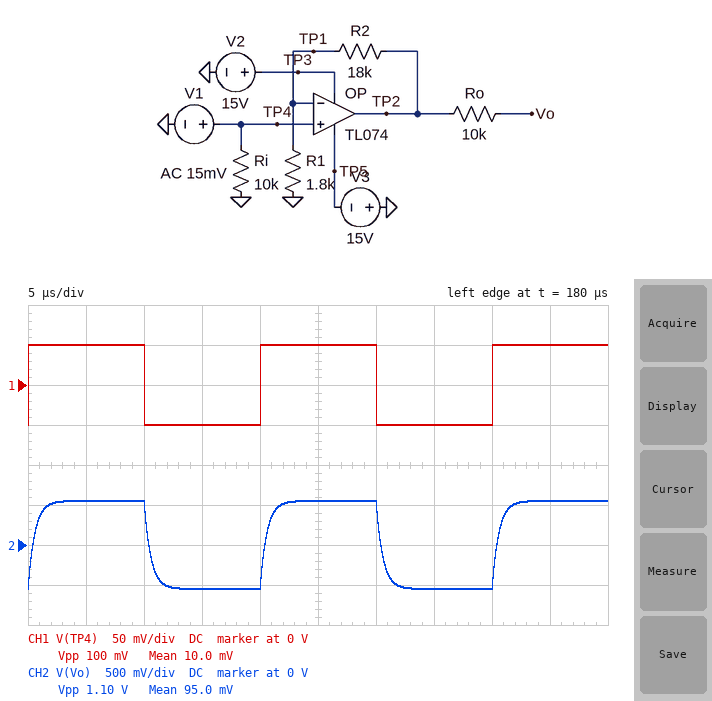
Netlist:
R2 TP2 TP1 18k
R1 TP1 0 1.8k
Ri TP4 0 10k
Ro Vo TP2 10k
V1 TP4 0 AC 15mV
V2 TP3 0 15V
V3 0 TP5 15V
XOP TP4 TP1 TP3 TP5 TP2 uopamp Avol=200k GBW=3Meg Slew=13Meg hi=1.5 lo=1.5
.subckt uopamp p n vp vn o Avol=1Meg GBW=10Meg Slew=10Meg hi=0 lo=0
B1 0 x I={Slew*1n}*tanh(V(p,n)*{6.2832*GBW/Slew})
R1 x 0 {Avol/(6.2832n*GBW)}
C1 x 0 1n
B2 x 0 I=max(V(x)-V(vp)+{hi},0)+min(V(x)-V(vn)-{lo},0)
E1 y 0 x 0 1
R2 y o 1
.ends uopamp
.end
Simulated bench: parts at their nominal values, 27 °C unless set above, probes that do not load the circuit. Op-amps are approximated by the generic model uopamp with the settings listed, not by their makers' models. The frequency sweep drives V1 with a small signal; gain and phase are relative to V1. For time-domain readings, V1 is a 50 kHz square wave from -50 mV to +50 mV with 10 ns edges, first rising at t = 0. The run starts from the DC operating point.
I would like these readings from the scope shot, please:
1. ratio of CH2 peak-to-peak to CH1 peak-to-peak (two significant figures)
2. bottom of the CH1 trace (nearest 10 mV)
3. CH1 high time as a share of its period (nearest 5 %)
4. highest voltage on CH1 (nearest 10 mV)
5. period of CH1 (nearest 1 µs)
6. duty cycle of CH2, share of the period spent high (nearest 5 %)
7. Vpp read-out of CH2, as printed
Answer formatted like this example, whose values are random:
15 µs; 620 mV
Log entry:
11; -50 mV; 50 %; 50 mV; 20 µs; 50 %; 1.10 V
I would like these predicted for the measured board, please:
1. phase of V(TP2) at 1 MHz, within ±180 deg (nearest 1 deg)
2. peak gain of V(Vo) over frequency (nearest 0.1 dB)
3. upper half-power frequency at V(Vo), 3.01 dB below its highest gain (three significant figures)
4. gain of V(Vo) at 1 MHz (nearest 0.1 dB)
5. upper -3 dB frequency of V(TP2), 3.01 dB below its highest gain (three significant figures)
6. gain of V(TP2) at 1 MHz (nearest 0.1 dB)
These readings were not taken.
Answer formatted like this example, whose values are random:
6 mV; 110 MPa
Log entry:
-75 deg; 20.8 dB; 273 kHz; 9.2 dB; 273 kHz; 9.2 dB
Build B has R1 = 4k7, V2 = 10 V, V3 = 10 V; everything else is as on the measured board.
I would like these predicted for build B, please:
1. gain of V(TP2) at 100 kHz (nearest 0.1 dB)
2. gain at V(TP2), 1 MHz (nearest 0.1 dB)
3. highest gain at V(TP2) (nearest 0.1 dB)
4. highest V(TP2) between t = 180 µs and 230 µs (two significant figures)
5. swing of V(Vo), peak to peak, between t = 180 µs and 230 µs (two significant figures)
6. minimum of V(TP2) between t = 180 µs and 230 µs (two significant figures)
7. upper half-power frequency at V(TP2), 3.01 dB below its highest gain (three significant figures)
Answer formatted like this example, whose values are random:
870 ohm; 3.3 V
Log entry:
13.6 dB; 8.1 dB; 13.7 dB; 240 mV; 480 mV; -240 mV; 621 kHz
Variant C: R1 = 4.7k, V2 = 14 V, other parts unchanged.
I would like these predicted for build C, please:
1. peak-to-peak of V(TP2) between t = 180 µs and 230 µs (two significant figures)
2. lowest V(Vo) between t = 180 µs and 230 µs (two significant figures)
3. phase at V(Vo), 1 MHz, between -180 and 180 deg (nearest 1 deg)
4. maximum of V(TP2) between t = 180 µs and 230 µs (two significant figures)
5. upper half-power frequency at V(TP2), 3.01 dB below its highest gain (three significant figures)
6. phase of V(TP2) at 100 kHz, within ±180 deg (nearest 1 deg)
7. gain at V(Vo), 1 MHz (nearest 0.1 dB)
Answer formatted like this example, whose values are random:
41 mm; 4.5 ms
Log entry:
480 mV; -240 mV; -58 deg; 240 mV; 621 kHz; -9 deg; 8.1 dB
